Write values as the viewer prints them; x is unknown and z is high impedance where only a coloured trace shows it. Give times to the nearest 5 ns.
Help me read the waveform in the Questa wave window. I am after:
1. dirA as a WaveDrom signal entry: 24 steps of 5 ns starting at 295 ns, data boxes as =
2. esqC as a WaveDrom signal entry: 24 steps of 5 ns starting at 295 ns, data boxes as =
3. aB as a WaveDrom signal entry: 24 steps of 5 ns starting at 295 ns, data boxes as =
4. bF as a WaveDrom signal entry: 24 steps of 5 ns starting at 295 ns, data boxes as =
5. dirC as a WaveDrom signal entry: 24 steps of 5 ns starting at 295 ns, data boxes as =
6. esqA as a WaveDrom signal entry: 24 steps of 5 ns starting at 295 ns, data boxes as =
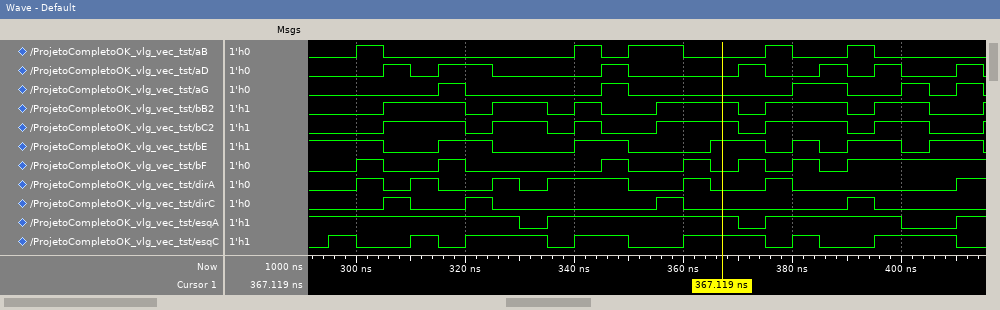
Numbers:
{name: 'dirA', wave: '01010.101..0.10.10.....1'}
{name: 'esqC', wave: '10.101..01.0.1..010.1..0'}
{name: 'aB', wave: '010......101.0..10.10...'}
{name: 'bF', wave: '010.10....10.1010101....'}
{name: 'dirC', wave: '0.10.10.....10.....10...'}
{name: 'esqA', wave: '1......01......01....0.1'}
